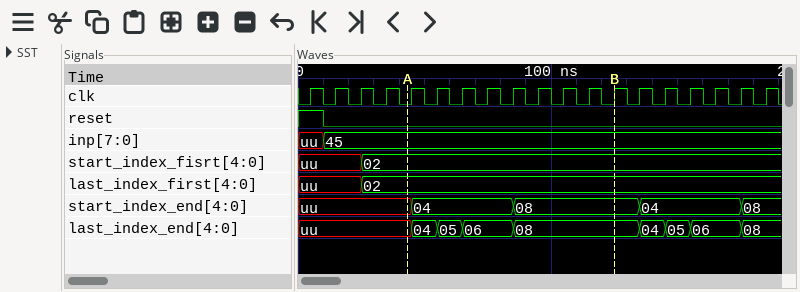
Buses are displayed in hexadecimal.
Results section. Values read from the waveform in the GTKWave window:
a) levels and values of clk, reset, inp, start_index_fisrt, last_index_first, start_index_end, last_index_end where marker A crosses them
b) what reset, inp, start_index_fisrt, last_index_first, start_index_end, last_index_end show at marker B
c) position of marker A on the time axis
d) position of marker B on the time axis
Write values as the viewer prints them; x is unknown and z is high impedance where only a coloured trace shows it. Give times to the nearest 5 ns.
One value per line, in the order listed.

clk=0, reset=0, inp=45, start_index_fisrt=02, last_index_first=02, start_index_end=uu, last_index_end=uu
reset=0, inp=45, start_index_fisrt=02, last_index_first=02, start_index_end=08, last_index_end=08
45 ns
125 ns
